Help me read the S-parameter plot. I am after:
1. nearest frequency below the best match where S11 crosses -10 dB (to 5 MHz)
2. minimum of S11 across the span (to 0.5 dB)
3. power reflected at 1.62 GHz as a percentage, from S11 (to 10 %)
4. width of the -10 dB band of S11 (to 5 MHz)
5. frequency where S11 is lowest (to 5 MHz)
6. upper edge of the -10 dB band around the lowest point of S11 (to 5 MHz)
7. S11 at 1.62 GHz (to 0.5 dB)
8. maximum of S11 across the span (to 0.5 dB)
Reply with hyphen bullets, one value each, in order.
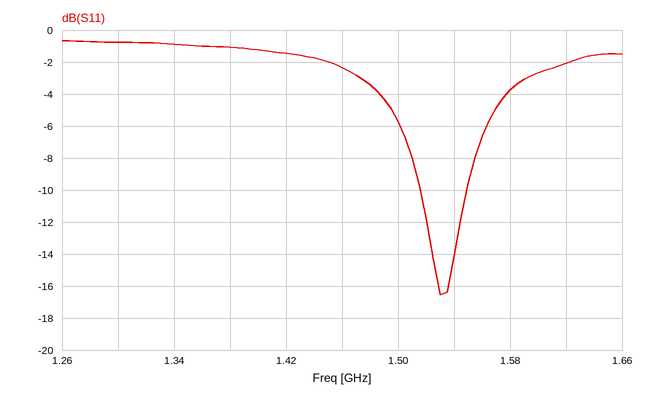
- 1.515 GHz
- -16.5 dB
- 60 %
- 35 MHz
- 1.530 GHz
- 1.550 GHz
- -2.0 dB
- -0.5 dB
